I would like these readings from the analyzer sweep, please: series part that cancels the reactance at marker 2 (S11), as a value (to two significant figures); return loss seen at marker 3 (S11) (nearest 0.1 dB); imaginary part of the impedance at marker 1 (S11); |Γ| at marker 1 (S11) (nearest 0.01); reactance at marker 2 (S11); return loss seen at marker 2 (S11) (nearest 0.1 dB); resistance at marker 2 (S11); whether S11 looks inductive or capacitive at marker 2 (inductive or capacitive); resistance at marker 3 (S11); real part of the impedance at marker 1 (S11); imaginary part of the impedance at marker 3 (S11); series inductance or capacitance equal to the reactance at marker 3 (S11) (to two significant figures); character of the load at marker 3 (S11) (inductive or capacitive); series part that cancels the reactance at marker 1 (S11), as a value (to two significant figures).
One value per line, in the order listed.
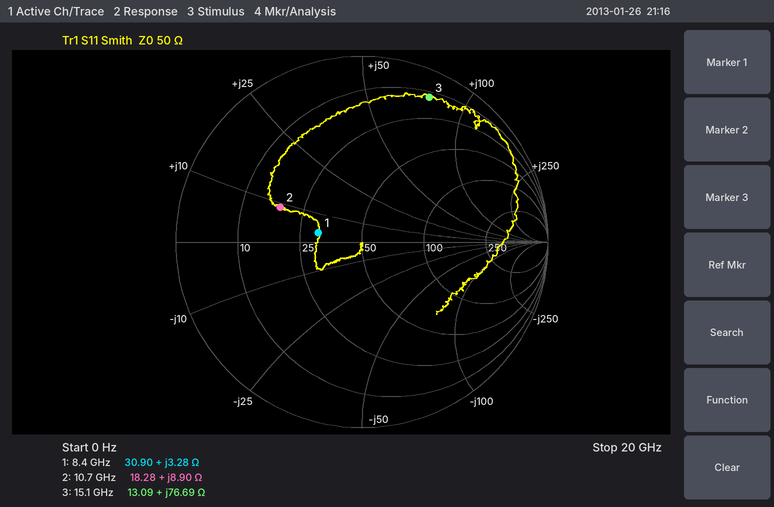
1.7 pF
1.3 dB
+3.28 Ω
0.24
+8.90 Ω
6.4 dB
18.28 Ω
inductive
13.09 Ω
30.90 Ω
+76.69 Ω
810 pH
inductive
5.8 pF
